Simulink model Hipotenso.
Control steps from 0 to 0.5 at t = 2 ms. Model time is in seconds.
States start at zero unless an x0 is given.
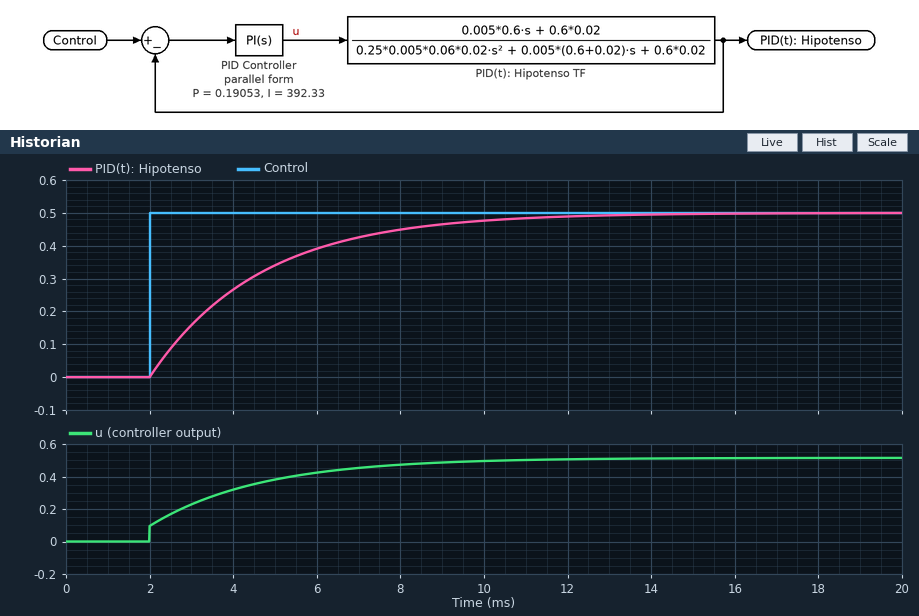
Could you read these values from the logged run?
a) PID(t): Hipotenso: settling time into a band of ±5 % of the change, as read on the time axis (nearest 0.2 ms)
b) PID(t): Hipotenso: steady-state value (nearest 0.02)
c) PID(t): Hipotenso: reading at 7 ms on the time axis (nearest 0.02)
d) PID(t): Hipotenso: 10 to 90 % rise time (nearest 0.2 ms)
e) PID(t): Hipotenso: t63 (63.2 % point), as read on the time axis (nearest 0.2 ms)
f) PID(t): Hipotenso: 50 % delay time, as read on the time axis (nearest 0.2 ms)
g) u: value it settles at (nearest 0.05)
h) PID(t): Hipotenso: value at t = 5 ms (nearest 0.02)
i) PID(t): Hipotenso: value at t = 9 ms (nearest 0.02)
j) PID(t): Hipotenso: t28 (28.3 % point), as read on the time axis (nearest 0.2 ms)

9.8 ms
0.50
0.42
5.8 ms
4.6 ms
3.8 ms
0.50
0.34
0.46
2.8 ms
